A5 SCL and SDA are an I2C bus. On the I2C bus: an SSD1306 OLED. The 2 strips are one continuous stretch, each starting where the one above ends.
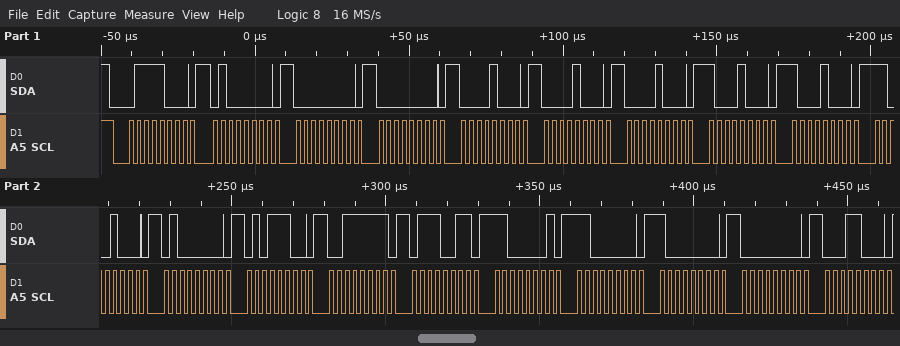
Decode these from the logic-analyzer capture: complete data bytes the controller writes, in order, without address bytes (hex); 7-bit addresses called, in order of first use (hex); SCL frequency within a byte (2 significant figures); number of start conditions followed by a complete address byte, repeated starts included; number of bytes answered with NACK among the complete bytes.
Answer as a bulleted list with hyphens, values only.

- 40 00 00 08 08 08 88 88 C8 40 5C 3F 73 C1 C0 80 00 18
- 0x3C
- 400 kHz
- 1
- 0
